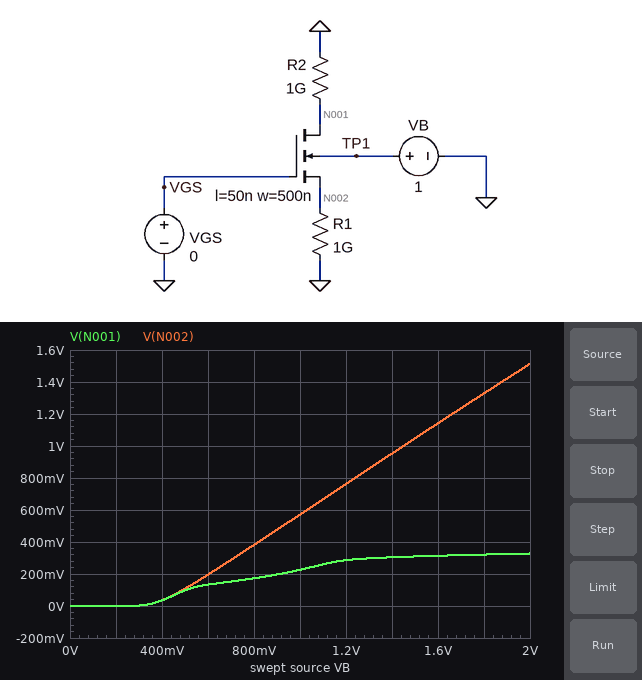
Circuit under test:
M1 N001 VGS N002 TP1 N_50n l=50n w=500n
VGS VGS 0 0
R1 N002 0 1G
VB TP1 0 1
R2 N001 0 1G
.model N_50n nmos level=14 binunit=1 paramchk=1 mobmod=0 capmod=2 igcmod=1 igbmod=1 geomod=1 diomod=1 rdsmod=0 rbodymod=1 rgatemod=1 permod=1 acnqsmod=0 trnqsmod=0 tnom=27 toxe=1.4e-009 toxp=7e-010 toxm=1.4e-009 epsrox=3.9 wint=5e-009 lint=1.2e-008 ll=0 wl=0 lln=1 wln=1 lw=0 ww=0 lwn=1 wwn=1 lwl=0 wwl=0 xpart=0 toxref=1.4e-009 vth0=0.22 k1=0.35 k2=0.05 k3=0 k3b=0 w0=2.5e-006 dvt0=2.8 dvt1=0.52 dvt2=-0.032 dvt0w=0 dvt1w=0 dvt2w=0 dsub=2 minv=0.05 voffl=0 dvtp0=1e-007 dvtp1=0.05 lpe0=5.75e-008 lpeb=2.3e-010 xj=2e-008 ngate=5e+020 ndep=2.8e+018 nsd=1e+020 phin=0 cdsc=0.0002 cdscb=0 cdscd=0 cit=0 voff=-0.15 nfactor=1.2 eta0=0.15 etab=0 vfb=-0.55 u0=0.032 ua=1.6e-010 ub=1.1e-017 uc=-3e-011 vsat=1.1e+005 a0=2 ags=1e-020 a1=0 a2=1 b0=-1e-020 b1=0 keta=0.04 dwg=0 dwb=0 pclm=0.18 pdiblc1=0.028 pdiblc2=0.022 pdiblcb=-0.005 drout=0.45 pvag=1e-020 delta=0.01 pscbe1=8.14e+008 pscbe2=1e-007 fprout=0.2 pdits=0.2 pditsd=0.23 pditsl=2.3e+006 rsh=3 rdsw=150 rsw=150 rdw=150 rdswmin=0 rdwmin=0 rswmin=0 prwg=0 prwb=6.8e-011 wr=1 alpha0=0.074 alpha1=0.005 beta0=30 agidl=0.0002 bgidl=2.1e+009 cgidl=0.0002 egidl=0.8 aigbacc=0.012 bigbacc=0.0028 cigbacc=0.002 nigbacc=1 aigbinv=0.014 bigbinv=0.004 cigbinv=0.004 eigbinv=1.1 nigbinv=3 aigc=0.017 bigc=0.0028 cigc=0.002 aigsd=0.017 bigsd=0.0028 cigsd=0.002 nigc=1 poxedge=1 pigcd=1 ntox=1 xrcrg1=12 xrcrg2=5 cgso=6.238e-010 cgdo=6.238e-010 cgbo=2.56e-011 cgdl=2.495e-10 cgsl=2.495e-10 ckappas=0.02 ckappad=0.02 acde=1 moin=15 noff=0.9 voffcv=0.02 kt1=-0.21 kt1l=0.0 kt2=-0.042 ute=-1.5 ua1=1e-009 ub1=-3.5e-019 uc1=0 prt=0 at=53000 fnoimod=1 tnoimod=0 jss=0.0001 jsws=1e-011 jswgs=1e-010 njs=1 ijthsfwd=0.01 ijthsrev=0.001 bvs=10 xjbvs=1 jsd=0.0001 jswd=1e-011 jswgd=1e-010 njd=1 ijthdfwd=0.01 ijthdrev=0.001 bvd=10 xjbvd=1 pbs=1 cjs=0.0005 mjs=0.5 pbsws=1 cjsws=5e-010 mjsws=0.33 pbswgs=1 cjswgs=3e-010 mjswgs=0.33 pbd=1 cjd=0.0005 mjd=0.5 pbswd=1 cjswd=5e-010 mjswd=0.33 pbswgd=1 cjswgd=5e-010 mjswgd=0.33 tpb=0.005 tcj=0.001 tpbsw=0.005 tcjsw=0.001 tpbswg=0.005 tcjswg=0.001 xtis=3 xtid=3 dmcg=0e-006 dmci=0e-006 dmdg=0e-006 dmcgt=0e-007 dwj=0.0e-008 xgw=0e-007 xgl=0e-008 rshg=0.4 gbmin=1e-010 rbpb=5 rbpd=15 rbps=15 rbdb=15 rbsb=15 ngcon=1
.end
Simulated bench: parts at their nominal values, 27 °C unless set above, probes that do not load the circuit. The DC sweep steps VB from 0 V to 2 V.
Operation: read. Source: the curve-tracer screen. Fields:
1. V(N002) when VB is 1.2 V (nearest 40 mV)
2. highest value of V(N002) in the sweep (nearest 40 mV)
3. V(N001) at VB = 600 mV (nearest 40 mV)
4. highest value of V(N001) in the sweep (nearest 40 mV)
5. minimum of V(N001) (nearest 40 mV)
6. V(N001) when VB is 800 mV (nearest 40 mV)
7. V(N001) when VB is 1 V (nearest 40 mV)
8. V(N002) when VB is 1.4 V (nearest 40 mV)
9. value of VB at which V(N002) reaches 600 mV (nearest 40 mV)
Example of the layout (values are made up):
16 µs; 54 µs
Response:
760 mV; 1.52 V; 120 mV; 320 mV; 0 V; 160 mV; 240 mV; 960 mV; 1.04 V
